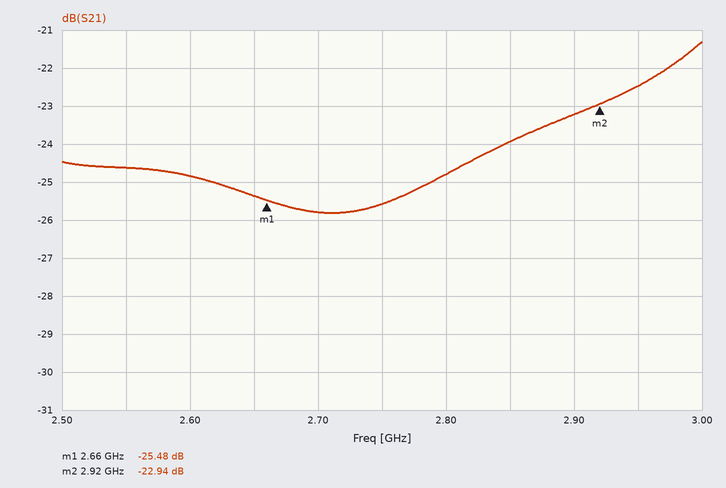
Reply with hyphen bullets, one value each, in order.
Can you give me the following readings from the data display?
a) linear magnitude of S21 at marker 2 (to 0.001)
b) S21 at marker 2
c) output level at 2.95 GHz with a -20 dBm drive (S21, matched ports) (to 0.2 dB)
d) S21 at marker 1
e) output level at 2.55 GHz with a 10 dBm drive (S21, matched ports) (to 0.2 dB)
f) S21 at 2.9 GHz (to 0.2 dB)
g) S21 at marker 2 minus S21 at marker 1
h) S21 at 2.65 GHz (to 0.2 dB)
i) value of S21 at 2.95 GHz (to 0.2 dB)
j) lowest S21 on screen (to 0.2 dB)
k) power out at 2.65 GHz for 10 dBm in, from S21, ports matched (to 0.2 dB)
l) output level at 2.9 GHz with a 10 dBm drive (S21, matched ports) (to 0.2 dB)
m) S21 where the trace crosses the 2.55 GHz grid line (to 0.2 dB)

- 0.071
- -22.94 dB
- -42.4 dBm
- -25.48 dB
- -14.6 dBm
- -23.2 dB
- 2.54 dB
- -25.4 dB
- -22.4 dB
- -25.8 dB
- -15.4 dBm
- -13.2 dBm
- -24.6 dB
